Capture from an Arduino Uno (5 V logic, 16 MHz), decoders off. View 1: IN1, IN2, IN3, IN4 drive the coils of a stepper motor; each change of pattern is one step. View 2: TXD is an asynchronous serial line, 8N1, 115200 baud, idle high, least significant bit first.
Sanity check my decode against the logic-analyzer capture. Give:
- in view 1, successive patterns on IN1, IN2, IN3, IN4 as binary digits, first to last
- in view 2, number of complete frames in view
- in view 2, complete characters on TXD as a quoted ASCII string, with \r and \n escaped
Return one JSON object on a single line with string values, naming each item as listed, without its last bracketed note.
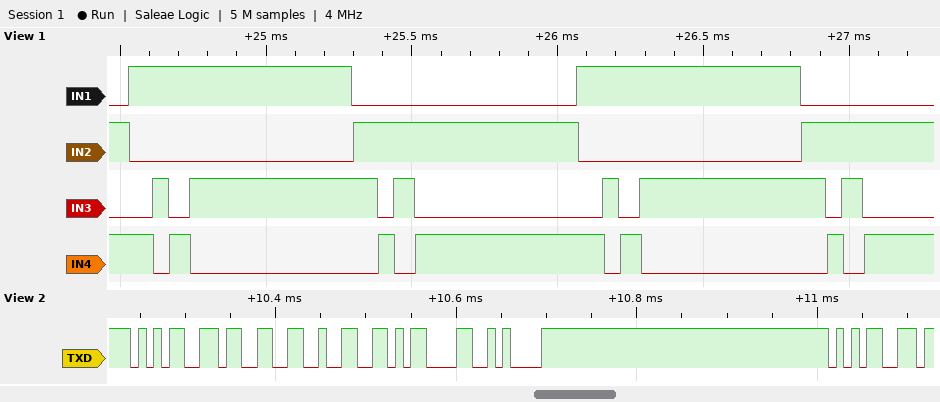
{"in view 1, successive patterns on IN1, IN2, IN3, IN4 as binary digits, first to last": "0101 1001 1001 1010 0110 0110 0101 1001 1001 1010 0110 0110 0101", "in view 2, number of complete frames in view": "6", "in view 2, complete characters on TXD as a quoted ASCII string, with \\r and \\n escaped": "\"532\\r\\n5\""}
